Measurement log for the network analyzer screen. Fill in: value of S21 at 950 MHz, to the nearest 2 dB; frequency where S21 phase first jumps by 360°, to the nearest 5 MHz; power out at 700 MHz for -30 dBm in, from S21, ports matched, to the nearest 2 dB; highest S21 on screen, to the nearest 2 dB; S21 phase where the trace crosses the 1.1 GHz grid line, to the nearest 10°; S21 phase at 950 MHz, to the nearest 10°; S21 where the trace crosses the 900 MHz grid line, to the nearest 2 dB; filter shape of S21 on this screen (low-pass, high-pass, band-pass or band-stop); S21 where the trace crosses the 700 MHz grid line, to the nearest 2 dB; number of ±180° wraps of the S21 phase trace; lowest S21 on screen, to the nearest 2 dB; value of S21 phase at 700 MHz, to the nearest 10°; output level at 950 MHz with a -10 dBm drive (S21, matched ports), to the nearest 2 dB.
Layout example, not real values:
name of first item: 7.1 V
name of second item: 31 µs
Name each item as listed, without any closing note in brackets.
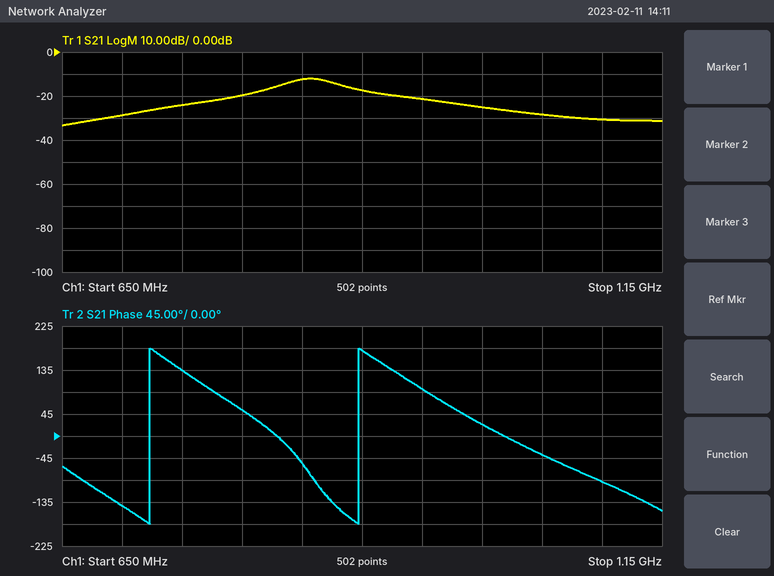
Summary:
value of S21 at 950 MHz, to the nearest 2 dB: -22 dB
frequency where S21 phase first jumps by 360°, to the nearest 5 MHz: 725 MHz
power out at 700 MHz for -30 dBm in, from S21, ports matched, to the nearest 2 dB: -58 dBm
highest S21 on screen, to the nearest 2 dB: -12 dB
S21 phase where the trace crosses the 1.1 GHz grid line, to the nearest 10°: -90°
S21 phase at 950 MHz, to the nearest 10°: 100°
S21 where the trace crosses the 900 MHz grid line, to the nearest 2 dB: -18 dB
filter shape of S21 on this screen: band-pass
S21 where the trace crosses the 700 MHz grid line, to the nearest 2 dB: -28 dB
number of ±180° wraps of the S21 phase trace: 2
lowest S21 on screen, to the nearest 2 dB: -34 dB
value of S21 phase at 700 MHz, to the nearest 10°: -140°
output level at 950 MHz with a -10 dBm drive (S21, matched ports), to the nearest 2 dB: -32 dBm
